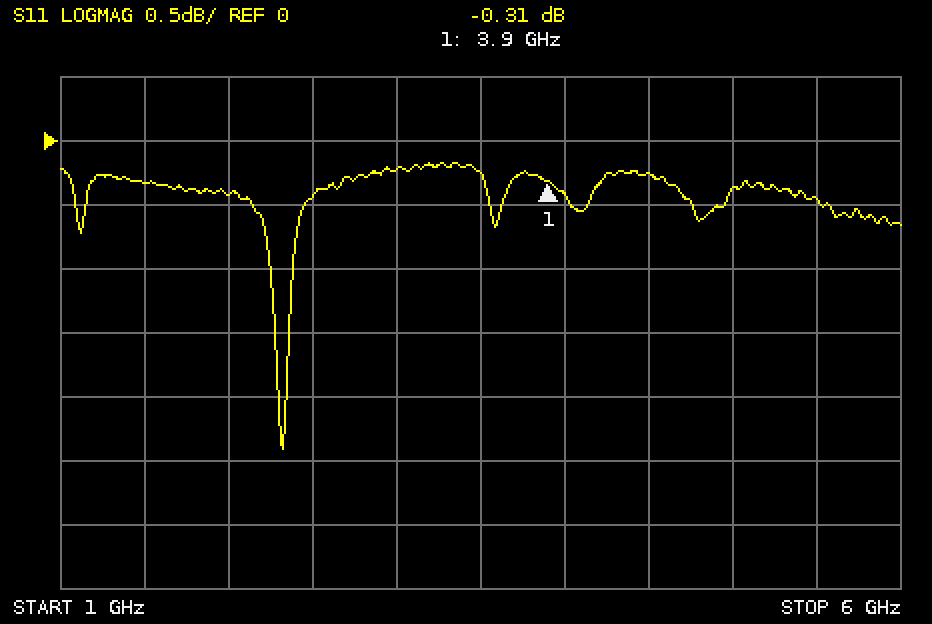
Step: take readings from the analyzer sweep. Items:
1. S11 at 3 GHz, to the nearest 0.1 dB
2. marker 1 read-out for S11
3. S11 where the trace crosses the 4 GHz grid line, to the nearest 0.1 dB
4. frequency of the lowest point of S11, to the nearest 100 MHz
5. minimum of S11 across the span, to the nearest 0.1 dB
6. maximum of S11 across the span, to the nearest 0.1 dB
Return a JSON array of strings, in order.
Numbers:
["-0.2 dB", "-0.31 dB", "-0.4 dB", "2.3 GHz", "-2.4 dB", "-0.2 dB"]
